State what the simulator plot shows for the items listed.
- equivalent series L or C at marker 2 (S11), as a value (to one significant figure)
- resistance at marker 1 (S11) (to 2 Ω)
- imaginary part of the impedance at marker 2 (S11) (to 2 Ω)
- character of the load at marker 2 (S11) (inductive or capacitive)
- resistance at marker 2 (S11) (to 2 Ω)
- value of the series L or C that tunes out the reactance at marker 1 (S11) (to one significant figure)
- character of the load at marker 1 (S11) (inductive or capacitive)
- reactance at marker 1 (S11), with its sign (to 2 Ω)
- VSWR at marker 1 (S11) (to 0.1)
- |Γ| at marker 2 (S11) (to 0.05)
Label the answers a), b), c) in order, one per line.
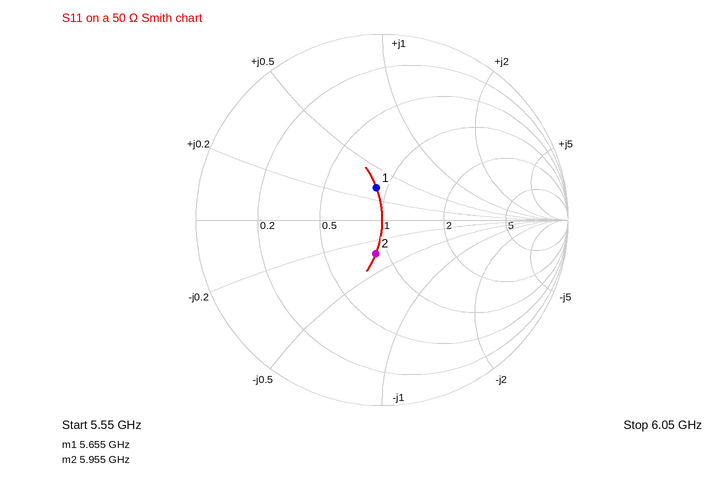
a) 2 pF
b) 44 Ω
c) -16 Ω
d) capacitive
e) 44 Ω
f) 2 pF
g) inductive
h) +16 Ω
i) 1.4
j) 0.20
